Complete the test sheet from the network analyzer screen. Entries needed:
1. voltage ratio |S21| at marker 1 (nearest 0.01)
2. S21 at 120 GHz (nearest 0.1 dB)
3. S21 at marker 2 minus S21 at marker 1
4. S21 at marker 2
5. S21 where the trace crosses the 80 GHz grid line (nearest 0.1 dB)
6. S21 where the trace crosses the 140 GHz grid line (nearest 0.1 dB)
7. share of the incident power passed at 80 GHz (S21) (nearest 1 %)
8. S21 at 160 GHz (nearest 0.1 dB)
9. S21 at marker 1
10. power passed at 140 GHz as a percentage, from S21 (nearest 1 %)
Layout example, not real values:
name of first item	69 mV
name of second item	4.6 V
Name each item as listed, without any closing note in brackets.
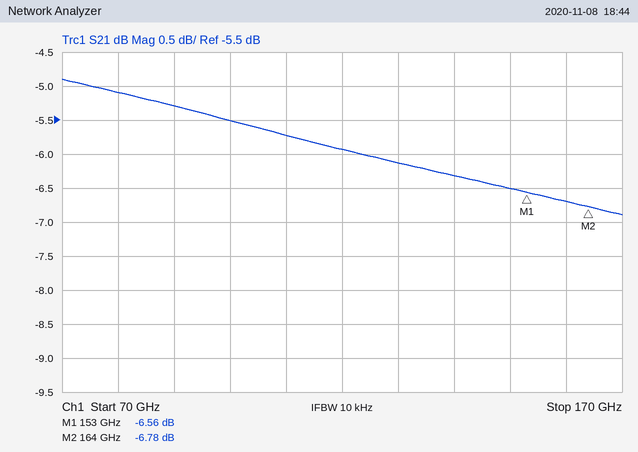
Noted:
voltage ratio |S21| at marker 1	0.47
S21 at 120 GHz	-5.9 dB
S21 at marker 2 minus S21 at marker 1	-0.22 dB
S21 at marker 2	-6.78 dB
S21 where the trace crosses the 80 GHz grid line	-5.1 dB
S21 where the trace crosses the 140 GHz grid line	-6.3 dB
share of the incident power passed at 80 GHz (S21)	31 %
S21 at 160 GHz	-6.7 dB
S21 at marker 1	-6.56 dB
power passed at 140 GHz as a percentage, from S21	23 %
